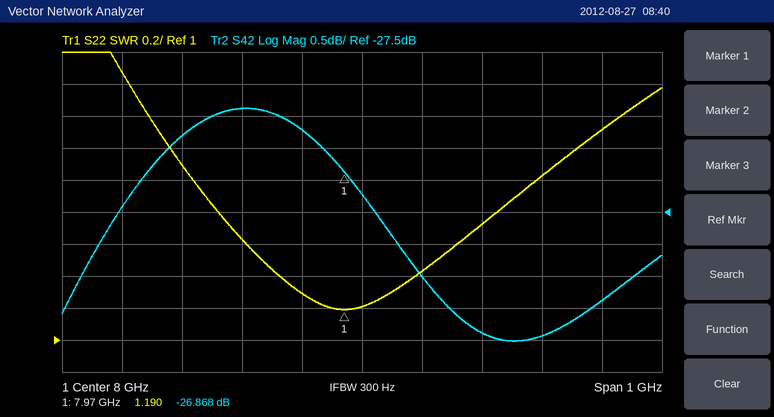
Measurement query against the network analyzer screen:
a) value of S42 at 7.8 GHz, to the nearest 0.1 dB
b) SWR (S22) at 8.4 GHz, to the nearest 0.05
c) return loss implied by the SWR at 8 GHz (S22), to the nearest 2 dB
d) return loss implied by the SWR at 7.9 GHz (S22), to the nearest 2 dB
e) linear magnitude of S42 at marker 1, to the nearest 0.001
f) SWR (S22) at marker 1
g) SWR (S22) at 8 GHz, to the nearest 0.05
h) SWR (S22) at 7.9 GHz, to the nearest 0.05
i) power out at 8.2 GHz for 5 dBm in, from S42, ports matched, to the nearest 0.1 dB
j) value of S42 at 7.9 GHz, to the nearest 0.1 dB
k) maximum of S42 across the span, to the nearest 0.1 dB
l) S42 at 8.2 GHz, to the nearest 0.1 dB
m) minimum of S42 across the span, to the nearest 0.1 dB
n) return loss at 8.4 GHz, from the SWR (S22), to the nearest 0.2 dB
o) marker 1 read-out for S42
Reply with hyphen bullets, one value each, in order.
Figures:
- -25.9 dB
- 2.30
- 20 dB
- 18 dB
- 0.045
- 1.190
- 1.20
- 1.30
- -24.4 dBm
- -26.2 dB
- -25.9 dB
- -29.4 dB
- -29.5 dB
- 8.0 dB
- -26.868 dB
